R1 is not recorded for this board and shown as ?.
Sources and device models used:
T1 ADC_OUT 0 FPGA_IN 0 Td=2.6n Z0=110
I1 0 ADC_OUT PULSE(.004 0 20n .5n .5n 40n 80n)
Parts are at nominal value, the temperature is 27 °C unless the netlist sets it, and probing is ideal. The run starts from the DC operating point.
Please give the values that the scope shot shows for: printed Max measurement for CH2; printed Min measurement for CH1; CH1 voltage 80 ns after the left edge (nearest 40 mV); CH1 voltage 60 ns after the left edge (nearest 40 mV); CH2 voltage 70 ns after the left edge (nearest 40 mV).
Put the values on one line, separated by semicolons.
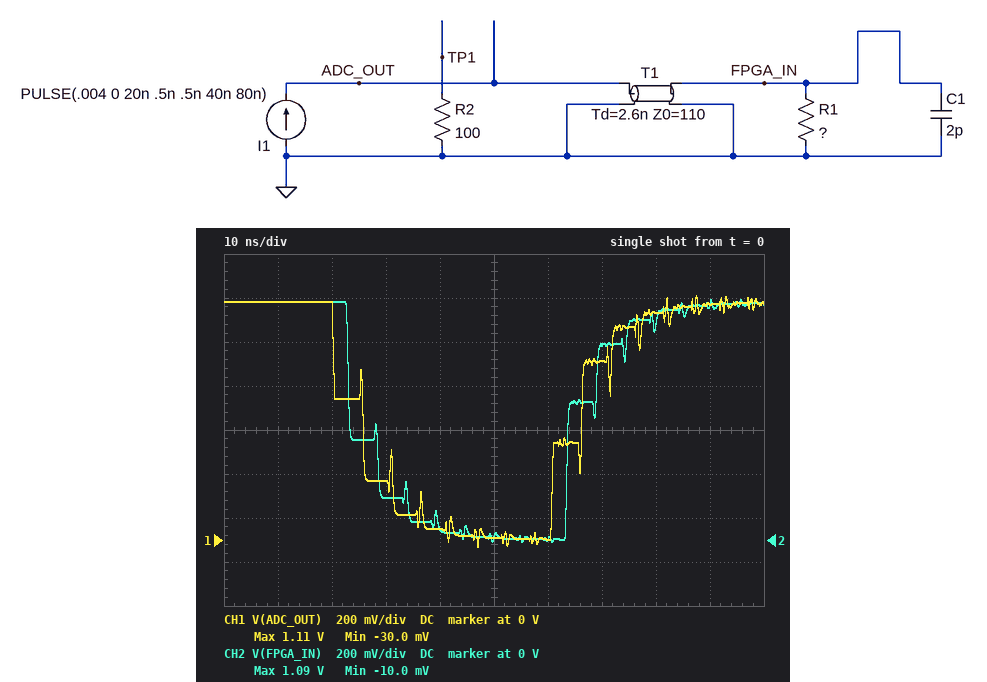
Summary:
1.09 V; -30.0 mV; 1.04 V; 0 V; 880 mV
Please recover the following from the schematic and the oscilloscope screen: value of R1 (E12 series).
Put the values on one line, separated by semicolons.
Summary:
270 Ω
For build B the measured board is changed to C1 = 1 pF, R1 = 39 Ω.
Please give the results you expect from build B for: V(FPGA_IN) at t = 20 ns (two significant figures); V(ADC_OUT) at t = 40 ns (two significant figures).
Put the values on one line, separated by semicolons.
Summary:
160 mV; 31 mV
